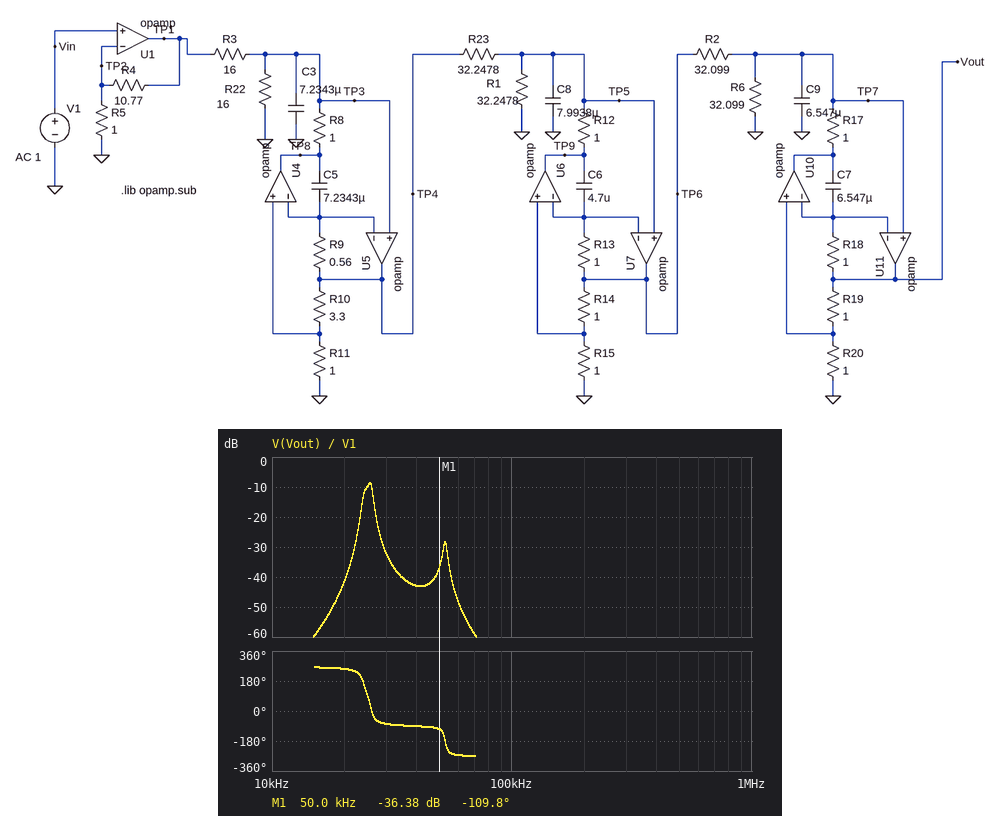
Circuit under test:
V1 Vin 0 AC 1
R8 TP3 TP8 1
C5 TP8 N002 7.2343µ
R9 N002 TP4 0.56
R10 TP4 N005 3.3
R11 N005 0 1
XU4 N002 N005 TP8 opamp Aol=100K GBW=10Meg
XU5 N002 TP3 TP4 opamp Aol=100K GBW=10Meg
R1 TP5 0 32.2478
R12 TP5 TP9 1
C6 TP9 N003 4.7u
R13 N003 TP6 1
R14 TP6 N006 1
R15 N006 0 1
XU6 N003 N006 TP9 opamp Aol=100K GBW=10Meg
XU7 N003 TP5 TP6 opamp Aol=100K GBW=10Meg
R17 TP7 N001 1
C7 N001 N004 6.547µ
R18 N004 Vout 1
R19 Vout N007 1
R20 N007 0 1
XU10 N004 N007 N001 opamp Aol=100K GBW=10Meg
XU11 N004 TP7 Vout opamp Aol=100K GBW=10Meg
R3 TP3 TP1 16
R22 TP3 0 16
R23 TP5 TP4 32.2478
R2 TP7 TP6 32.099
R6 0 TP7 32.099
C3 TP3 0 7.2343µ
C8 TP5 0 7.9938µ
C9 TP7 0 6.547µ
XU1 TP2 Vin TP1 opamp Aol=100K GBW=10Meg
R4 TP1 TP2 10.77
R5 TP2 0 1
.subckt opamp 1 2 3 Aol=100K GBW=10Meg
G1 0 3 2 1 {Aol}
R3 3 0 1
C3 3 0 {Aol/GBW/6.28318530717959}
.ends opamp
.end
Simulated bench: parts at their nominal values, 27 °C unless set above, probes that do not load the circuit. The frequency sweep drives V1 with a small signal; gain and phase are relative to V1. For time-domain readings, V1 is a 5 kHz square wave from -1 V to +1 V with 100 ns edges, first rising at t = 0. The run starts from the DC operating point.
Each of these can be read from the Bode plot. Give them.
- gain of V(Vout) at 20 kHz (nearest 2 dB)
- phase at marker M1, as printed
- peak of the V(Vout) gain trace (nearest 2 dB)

-42 dB
-109.8 deg
-8 dB
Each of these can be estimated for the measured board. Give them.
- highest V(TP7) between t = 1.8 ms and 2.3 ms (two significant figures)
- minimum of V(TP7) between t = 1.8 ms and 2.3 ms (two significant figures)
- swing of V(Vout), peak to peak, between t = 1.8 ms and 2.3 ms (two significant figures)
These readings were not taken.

42 mV
-42 mV
170 mV
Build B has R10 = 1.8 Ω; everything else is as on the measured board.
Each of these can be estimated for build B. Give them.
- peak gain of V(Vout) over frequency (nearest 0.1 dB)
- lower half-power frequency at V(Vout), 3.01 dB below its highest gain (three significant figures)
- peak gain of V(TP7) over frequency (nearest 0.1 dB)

-4.6 dB
24.3 kHz
-10.6 dB
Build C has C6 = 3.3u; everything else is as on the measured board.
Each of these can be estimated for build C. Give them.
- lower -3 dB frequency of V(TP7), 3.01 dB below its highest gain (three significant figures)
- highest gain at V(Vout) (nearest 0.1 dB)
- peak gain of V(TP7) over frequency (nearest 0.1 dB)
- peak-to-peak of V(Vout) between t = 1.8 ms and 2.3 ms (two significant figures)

30.1 kHz
-16.8 dB
-22.8 dB
33 mV
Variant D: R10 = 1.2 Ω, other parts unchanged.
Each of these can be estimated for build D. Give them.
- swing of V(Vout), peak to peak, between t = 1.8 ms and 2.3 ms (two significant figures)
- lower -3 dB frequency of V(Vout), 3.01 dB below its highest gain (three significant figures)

460 mV
24.5 kHz
